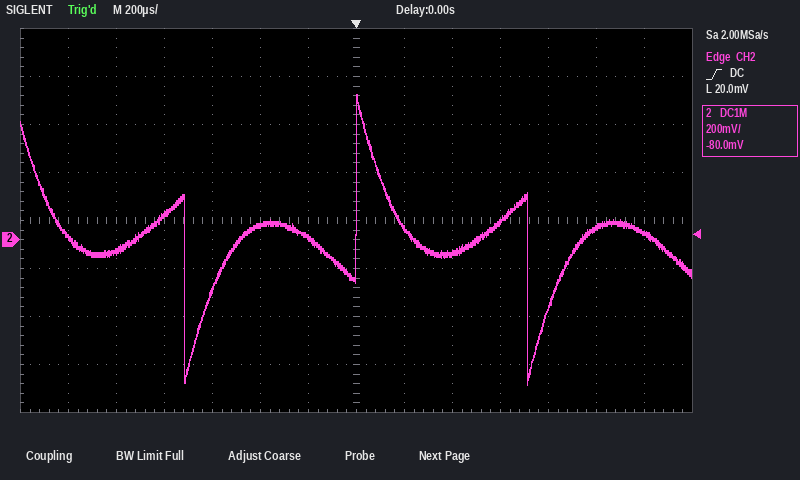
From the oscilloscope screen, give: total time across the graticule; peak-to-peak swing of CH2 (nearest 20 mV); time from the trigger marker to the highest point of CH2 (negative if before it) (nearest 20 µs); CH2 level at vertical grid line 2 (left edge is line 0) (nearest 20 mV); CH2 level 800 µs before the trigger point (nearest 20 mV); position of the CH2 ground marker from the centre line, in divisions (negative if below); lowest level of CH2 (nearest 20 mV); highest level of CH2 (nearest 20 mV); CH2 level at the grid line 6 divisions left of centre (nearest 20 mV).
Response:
2.8 ms
1.20 V
0 µs
-40 mV
100 mV
-0.4 div
-600 mV
600 mV
20 mV
